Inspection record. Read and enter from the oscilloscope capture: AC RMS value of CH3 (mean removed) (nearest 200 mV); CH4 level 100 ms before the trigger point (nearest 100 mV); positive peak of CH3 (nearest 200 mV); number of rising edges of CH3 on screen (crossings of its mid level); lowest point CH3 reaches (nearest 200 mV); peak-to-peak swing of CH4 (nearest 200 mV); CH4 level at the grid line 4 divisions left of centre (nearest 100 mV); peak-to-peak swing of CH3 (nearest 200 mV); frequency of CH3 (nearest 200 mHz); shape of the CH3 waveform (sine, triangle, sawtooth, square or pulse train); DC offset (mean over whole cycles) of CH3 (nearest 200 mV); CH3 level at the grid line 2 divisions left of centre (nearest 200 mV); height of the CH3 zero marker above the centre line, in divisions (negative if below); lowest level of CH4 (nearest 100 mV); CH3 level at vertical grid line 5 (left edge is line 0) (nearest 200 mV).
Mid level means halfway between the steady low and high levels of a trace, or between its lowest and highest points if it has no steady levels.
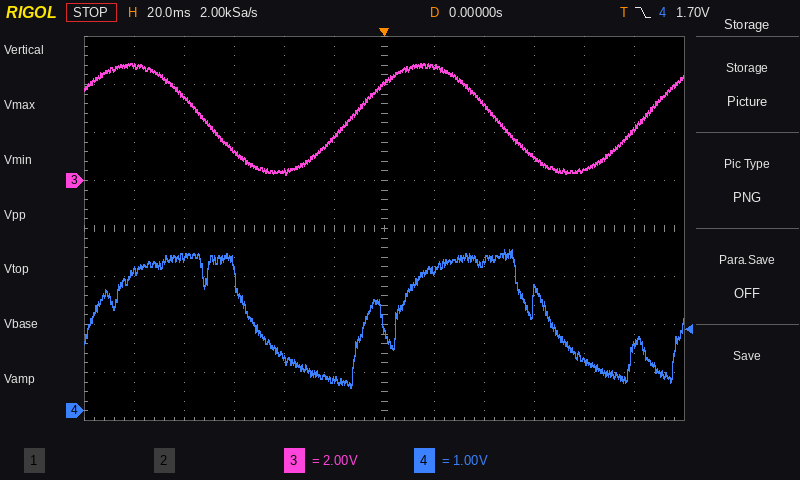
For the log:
1.6 V
2.9 V
4.8 V
2
200 mV
2.8 V
3.2 V
4.6 V
8.6 Hz
sine
2.6 V
400 mV
+1.0 div
500 mV
1.8 V
